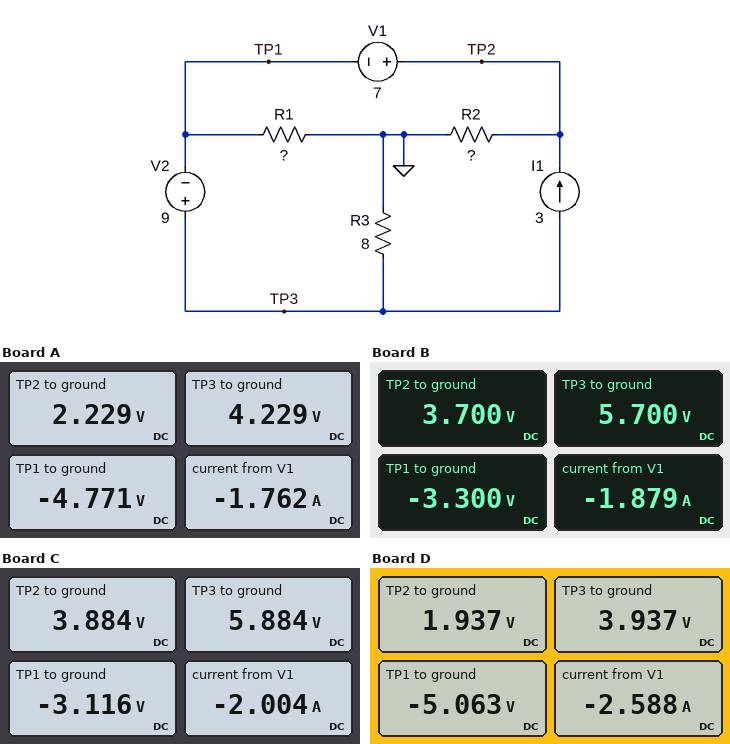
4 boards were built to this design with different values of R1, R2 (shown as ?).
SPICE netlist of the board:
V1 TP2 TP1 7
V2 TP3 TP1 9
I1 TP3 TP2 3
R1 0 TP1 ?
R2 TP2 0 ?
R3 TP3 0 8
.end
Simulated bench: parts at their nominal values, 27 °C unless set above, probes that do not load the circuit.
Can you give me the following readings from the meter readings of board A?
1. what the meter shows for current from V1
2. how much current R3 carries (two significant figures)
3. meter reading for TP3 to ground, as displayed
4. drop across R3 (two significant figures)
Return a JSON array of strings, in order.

["-1.762 A", "530 mA", "4.229 V", "4.2 V"]
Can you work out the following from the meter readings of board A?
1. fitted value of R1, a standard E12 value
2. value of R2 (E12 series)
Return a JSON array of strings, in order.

["2.7 Ω", "1.8 Ω"]
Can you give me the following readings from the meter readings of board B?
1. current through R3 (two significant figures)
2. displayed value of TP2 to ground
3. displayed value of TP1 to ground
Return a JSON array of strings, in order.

["710 mA", "3.700 V", "-3.300 V"]
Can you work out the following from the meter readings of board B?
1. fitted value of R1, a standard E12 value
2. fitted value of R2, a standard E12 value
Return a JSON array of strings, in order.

["1.8 Ω", "3.3 Ω"]
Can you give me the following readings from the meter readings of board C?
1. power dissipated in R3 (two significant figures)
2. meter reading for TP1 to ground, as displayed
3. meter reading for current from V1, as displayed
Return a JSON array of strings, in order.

["4.3 W", "-3.116 V", "-2.004 A"]
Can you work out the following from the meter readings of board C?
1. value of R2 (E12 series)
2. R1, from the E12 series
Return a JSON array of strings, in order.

["3.9 Ω", "1.8 Ω"]
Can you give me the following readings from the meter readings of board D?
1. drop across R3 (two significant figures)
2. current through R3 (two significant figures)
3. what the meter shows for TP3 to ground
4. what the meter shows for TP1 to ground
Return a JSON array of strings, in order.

["3.9 V", "490 mA", "3.937 V", "-5.063 V"]
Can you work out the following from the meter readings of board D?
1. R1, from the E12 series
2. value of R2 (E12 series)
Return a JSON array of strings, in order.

["5.6 Ω", "4.7 Ω"]
